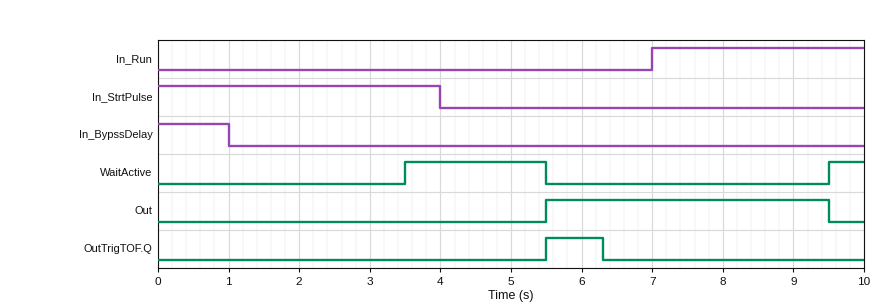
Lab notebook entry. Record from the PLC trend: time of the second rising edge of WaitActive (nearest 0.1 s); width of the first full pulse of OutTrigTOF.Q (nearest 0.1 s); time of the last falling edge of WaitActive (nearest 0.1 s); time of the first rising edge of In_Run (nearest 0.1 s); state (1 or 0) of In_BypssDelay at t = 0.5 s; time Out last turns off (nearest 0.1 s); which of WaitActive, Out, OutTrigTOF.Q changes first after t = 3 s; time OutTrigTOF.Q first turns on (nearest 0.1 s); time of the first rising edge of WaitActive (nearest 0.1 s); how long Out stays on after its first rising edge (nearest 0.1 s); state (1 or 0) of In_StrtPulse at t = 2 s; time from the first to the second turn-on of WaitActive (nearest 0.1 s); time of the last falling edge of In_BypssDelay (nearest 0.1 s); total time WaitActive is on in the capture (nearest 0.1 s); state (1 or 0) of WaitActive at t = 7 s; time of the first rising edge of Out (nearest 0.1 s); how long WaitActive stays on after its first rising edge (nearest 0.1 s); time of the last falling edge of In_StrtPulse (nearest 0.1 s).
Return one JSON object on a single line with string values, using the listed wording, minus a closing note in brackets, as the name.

{"time of the second rising edge of WaitActive": "9.5 s", "width of the first full pulse of OutTrigTOF.Q": "0.8 s", "time of the last falling edge of WaitActive": "5.5 s", "time of the first rising edge of In_Run": "7.0 s", "state (1 or 0) of In_BypssDelay at t = 0.5 s": "1", "time Out last turns off": "9.5 s", "which of WaitActive, Out, OutTrigTOF.Q changes first after t = 3 s": "WaitActive", "time OutTrigTOF.Q first turns on": "5.5 s", "time of the first rising edge of WaitActive": "3.5 s", "how long Out stays on after its first rising edge": "4.0 s", "state (1 or 0) of In_StrtPulse at t = 2 s": "1", "time from the first to the second turn-on of WaitActive": "6.0 s", "time of the last falling edge of In_BypssDelay": "1.0 s", "total time WaitActive is on in the capture": "2.5 s", "state (1 or 0) of WaitActive at t = 7 s": "0", "time of the first rising edge of Out": "5.5 s", "how long WaitActive stays on after its first rising edge": "2.0 s", "time of the last falling edge of In_StrtPulse": "4.0 s"}
